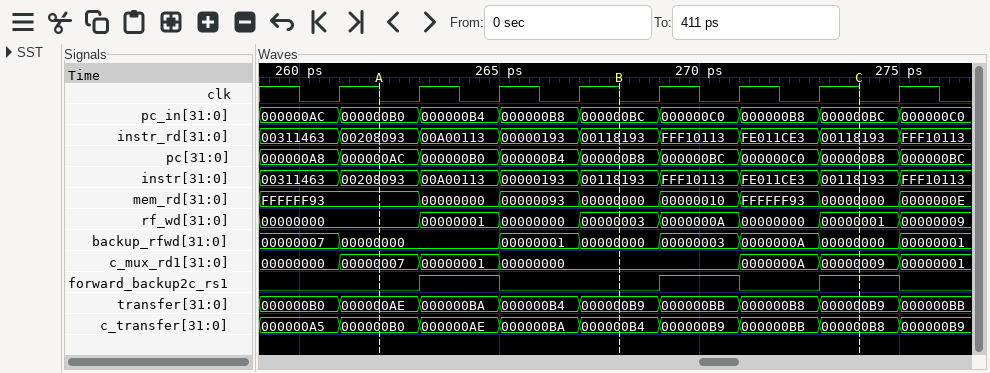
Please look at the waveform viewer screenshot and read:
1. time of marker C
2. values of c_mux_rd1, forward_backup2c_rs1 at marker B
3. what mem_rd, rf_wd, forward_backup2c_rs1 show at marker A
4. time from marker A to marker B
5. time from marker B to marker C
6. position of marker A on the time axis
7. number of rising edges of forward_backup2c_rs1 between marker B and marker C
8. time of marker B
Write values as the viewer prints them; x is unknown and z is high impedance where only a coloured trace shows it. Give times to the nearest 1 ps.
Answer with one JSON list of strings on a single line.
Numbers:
["274 ps", "c_mux_rd1=00000000, forward_backup2c_rs1=0", "mem_rd=FFFFFF93, rf_wd=00000000, forward_backup2c_rs1=0", "6 ps", "6 ps", "262 ps", "2", "268 ps"]
